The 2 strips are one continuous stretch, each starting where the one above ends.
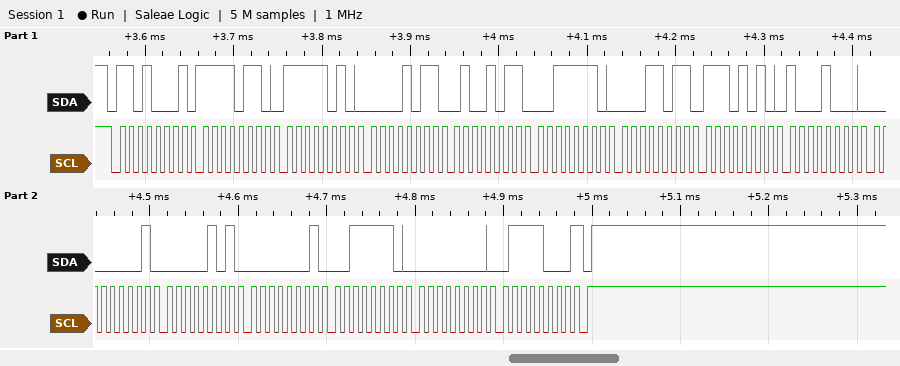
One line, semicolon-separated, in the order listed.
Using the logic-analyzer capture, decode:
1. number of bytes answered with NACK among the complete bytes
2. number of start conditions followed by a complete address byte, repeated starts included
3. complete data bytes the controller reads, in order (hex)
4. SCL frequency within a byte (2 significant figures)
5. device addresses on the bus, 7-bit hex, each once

1; 1; F6 FA 0B 4B 3E 1B EA 88 01 05 01 3E 00 78; 100 kHz; 0x68
